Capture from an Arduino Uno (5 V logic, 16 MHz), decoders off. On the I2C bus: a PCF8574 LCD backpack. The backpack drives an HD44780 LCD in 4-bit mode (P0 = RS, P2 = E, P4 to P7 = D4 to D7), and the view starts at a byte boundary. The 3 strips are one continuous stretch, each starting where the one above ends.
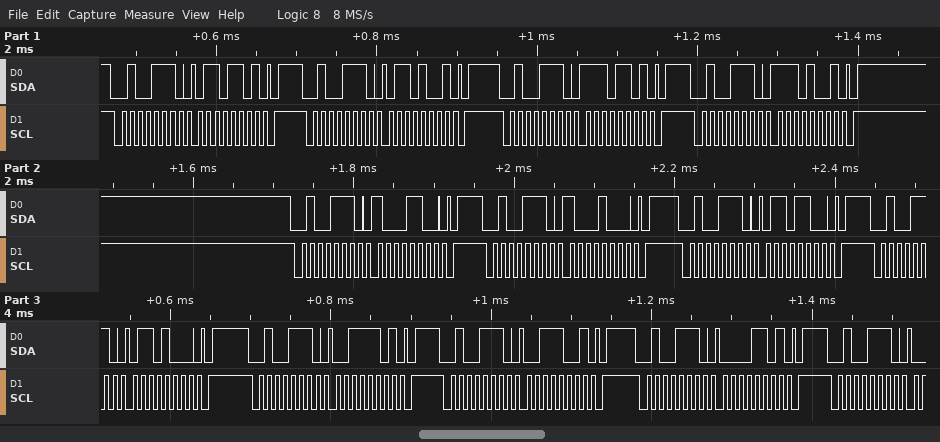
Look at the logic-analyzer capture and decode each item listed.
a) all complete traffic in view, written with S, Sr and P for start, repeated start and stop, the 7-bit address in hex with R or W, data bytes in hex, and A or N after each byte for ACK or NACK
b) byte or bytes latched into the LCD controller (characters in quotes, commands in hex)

S 27W A 6D A P S 27W A 69 A P S 27W A ED A P S 27W A E9 A P S 27W A 8C A P S 27W A 88 A P S 27W A 6C A P S 27W A 68 A P S 27W A 3D A P S 27W A 39 A P S 27W A 0D A P S 27W A
'n' 0x86
